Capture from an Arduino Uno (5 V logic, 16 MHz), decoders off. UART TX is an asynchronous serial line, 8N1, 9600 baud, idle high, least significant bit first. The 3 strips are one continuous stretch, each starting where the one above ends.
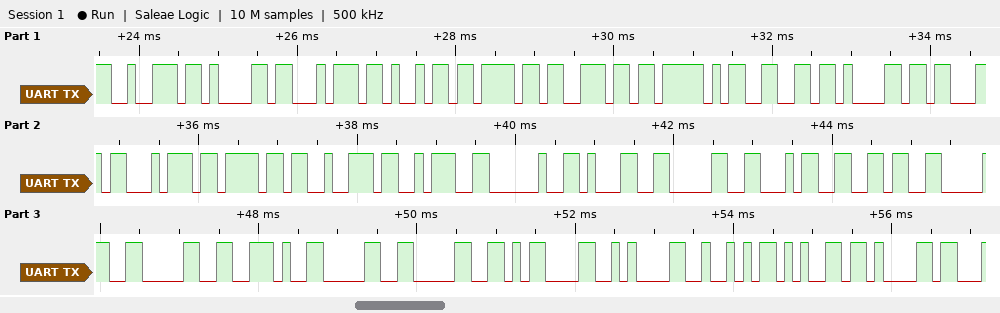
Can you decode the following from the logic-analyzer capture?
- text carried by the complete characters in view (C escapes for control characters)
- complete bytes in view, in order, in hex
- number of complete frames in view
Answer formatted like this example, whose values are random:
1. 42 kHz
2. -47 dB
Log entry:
1. "ration_factor: 104600.00\r\nRea"
2. 0x72 0x61 0x74 0x69 0x6F 0x6E 0x5F 0x66 0x61 0x63 0x74 0x6F 0x72 0x3A 0x20 0x31 0x30 0x34 0x36 0x30 0x30 0x2E 0x30 0x30 0x0D 0x0A 0x52 0x65 0x61
3. 29
